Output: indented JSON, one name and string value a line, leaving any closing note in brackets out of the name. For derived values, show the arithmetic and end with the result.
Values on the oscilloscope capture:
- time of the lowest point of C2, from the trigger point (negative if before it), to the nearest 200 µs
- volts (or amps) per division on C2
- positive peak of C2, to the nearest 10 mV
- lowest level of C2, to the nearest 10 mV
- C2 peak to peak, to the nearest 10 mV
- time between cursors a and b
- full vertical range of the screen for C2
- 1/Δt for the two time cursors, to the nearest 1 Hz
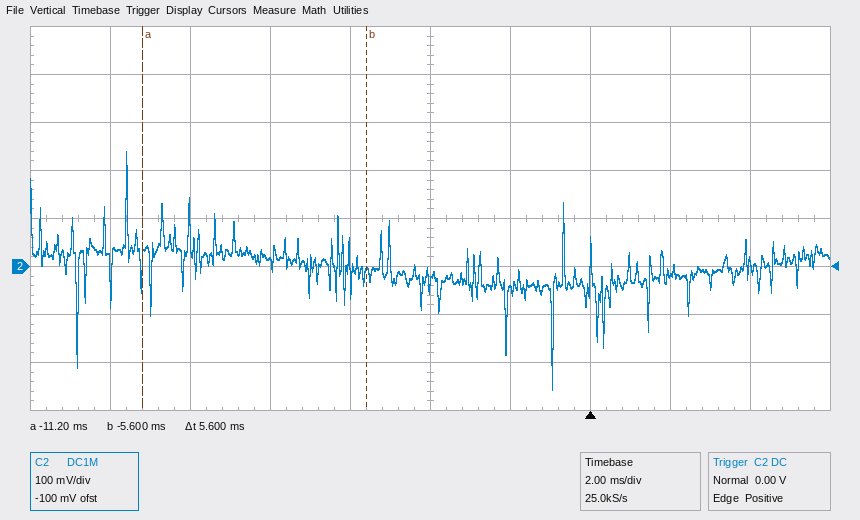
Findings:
{
  "time of the lowest point of C2, from the trigger point (negative if before it), to the nearest 200 µs": "-1.0 ms",
  "volts (or amps) per division on C2": "100 mV",
  "positive peak of C2, to the nearest 10 mV": "240 mV",
  "lowest level of C2, to the nearest 10 mV": "-260 mV",
  "C2 peak to peak, to the nearest 10 mV": "240 mV − (-260 mV) = 500 mV",
  "time between cursors a and b": "5.6 ms",
  "full vertical range of the screen for C2": "800 mV",
  "1/Δt for the two time cursors, to the nearest 1 Hz": "1 / 5.6 ms ≈ 179 Hz"
}
